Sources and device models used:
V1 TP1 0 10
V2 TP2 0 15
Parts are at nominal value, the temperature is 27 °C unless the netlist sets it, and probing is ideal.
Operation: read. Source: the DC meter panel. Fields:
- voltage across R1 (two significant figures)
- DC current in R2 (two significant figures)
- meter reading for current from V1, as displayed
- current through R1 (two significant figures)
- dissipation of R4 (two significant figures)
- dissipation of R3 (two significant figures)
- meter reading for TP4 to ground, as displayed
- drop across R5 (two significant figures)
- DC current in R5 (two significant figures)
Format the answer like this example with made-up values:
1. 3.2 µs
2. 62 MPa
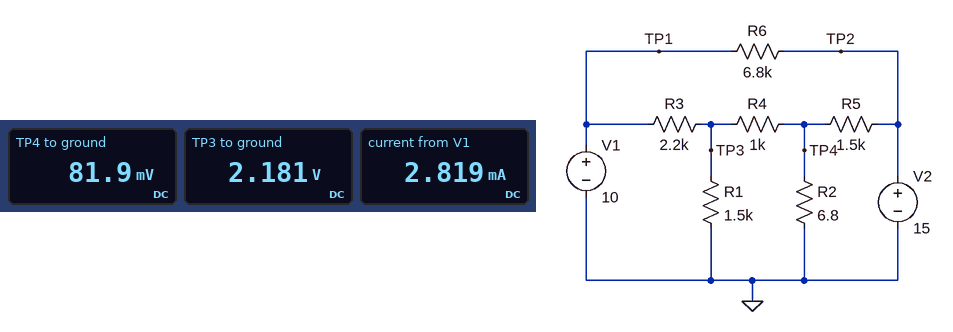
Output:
1. 2.2 V
2. 12 mA
3. 2.819 mA
4. 1.5 mA
5. 4.4 mW
6. 28 mW
7. 81.9 mV
8. 15 V
9. 9.9 mA
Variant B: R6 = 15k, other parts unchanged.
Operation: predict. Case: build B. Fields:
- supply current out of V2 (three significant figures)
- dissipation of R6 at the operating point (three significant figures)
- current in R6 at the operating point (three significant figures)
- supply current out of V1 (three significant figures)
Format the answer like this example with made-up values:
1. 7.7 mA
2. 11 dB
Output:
1. 10.3 mA
2. 1.67 mW
3. 333 µA
4. 3.22 mA
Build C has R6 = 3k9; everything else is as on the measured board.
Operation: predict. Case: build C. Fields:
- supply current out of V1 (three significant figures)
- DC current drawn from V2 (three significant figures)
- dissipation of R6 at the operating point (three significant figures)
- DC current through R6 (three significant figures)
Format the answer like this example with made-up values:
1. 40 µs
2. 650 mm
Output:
1. 2.27 mA
2. 11.2 mA
3. 6.41 mW
4. 1.28 mA
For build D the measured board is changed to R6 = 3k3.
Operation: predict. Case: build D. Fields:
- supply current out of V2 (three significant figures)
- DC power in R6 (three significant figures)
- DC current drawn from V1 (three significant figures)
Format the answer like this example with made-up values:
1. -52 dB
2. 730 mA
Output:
1. 11.5 mA
2. 7.58 mW
3. 2.04 mA
